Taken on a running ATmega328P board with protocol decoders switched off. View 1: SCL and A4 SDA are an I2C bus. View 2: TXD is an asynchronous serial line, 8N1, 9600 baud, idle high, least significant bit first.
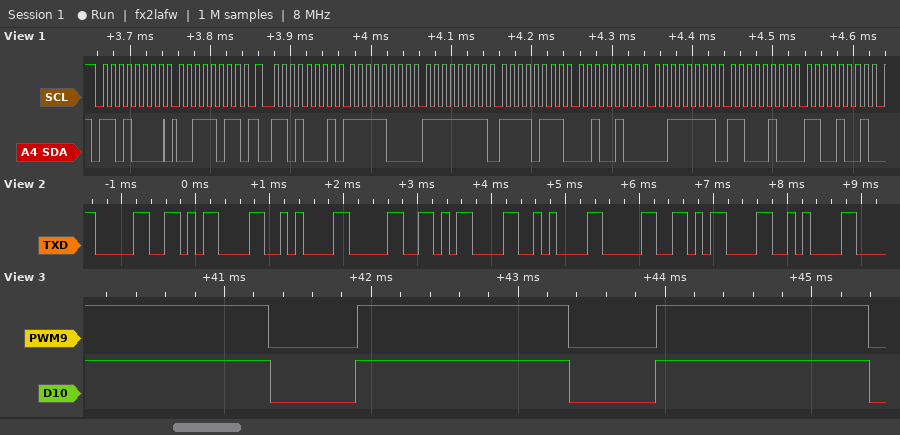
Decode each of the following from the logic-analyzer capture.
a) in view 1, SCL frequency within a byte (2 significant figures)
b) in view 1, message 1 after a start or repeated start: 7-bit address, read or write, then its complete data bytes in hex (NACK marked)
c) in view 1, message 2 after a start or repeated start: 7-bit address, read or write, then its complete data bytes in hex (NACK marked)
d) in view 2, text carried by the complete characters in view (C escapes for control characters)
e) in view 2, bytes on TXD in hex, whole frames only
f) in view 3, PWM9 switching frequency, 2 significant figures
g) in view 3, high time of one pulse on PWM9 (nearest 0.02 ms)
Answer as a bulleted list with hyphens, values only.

- 100 kHz
- 0x68 write: 3B
- 0x68 read: F8 FF F7 24 3F C4 C9
- "0\r\n0\r\n0\r\n"
- 30 0D 0A 30 0D 0A 30 0D 0A
- 490 Hz
- 1.44 ms
